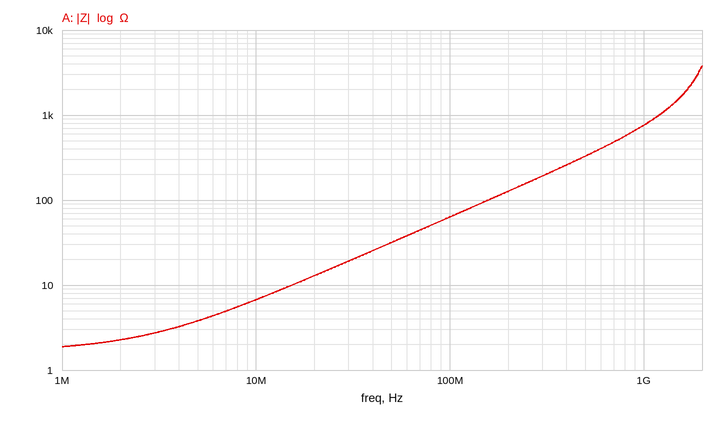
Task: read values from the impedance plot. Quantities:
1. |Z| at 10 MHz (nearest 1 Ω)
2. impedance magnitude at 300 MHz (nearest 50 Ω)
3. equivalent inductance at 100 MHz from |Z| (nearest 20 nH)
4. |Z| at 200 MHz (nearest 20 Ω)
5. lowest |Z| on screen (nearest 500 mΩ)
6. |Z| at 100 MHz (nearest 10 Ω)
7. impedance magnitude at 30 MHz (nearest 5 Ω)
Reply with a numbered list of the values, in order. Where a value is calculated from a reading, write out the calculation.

1. 7 Ω
2. 200 Ω
3. L = 60 Ω/(2π × 100 MHz) ≈ 95.5 nH, so 100 nH to the nearest 20 nH
4. 120 Ω
5. 2.0 Ω
6. 60 Ω
7. 20 Ω
